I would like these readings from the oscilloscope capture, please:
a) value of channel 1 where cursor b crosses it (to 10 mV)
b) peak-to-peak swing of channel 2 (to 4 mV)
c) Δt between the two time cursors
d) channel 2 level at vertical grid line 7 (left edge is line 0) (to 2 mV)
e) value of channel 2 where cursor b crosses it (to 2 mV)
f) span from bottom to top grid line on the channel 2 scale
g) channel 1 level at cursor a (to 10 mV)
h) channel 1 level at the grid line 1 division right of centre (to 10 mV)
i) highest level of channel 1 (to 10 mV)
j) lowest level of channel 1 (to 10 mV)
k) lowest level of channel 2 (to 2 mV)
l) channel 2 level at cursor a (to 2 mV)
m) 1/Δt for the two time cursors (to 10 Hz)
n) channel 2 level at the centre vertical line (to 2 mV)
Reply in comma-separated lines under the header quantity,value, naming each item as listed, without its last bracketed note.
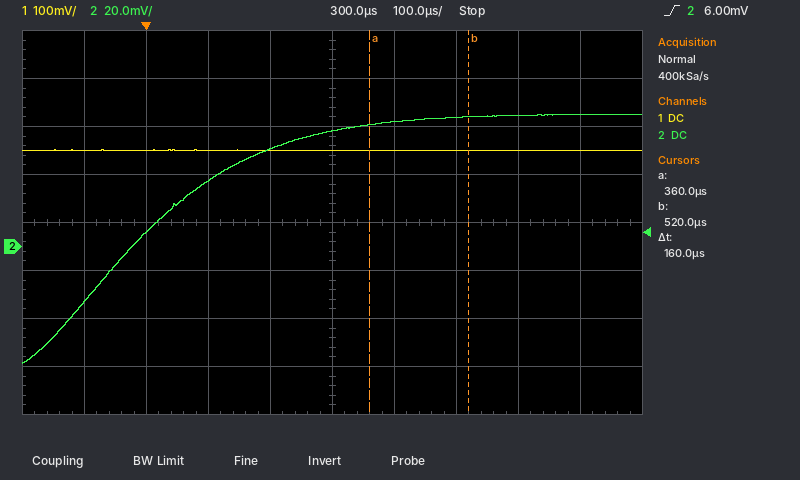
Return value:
quantity,value
value of channel 1 where cursor b crosses it,200 mV
peak-to-peak swing of channel 2,104 mV
Δt between the two time cursors,160 µs
channel 2 level at vertical grid line 7 (left edge is line 0),54 mV
value of channel 2 where cursor b crosses it,54 mV
span from bottom to top grid line on the channel 2 scale,160 mV
channel 1 level at cursor a,200 mV
channel 1 level at the grid line 1 division right of centre,200 mV
highest level of channel 1,200 mV
lowest level of channel 1,200 mV
lowest level of channel 2,-48 mV
channel 2 level at cursor a,50 mV
1/Δt for the two time cursors,6.25 kHz
channel 2 level at the centre vertical line,48 mV
